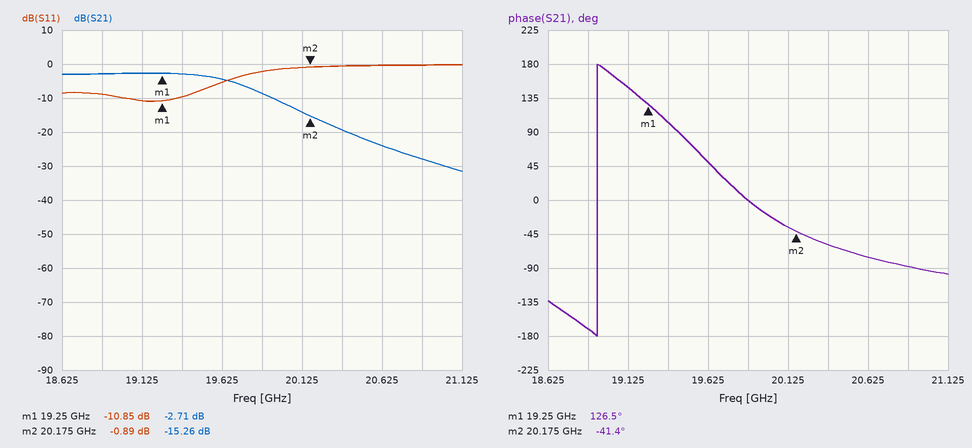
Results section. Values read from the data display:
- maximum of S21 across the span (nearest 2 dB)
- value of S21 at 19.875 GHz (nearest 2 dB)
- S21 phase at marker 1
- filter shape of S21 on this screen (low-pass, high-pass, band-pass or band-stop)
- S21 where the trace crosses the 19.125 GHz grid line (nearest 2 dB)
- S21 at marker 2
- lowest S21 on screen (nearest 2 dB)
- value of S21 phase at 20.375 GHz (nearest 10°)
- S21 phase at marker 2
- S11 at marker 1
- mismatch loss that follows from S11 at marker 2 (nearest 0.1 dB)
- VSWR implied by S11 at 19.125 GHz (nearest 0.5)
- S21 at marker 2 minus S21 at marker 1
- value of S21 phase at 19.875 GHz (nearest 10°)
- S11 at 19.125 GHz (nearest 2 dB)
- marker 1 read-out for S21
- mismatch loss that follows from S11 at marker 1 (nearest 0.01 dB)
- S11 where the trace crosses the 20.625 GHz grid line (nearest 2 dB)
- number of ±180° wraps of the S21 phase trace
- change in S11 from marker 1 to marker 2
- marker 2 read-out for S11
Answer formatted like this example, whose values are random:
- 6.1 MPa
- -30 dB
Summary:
- -2 dB
- -8 dB
- 126.5°
- low-pass
- -2 dB
- -15.26 dB
- -32 dB
- -60°
- -41.4°
- -10.85 dB
- 7.3 dB
- 2.0
- -12.55 dB
- 0°
- -10 dB
- -2.71 dB
- 0.37 dB
- 0 dB
- 1
- 9.96 dB
- -0.89 dB
